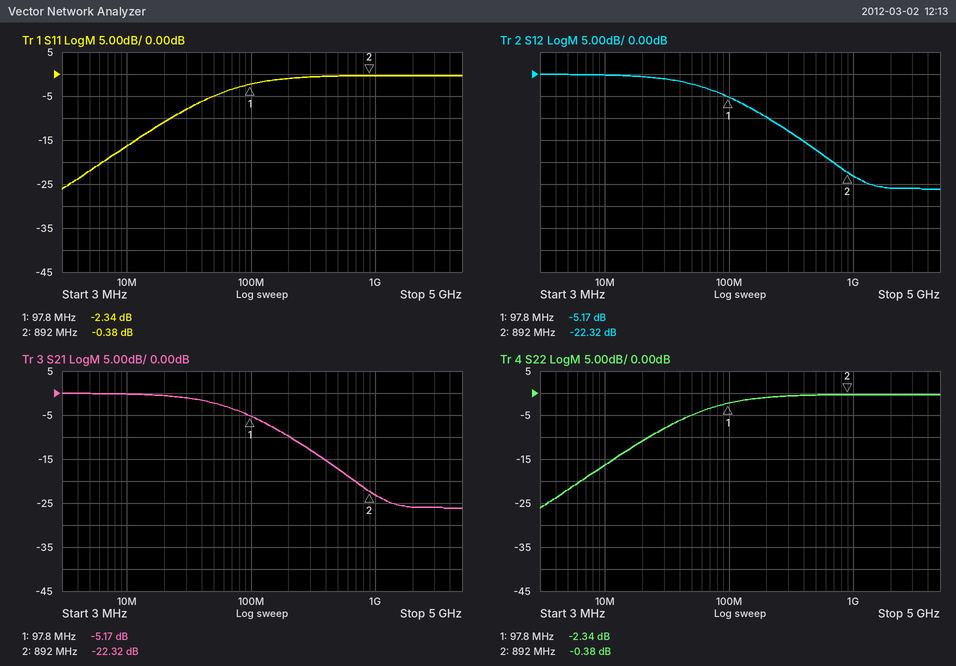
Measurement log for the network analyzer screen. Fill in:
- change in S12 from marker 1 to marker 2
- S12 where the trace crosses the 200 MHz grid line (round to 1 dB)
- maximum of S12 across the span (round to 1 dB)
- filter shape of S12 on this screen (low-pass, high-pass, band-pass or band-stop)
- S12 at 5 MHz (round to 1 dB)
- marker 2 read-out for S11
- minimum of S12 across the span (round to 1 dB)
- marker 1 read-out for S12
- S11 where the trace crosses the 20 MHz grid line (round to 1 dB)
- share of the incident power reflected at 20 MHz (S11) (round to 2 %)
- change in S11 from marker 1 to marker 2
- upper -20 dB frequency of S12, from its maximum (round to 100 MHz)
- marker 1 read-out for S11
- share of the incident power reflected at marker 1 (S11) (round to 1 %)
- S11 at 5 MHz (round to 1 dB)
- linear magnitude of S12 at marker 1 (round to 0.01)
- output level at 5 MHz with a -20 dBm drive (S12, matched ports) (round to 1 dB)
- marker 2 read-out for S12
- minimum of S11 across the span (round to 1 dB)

-17.15 dB
-10 dB
0 dB
low-pass
0 dB
-0.38 dB
-26 dB
-5.17 dB
-11 dB
8 %
1.96 dB
700 MHz
-2.34 dB
58 %
-22 dB
0.55
-20 dBm
-22.32 dB
-26 dB
